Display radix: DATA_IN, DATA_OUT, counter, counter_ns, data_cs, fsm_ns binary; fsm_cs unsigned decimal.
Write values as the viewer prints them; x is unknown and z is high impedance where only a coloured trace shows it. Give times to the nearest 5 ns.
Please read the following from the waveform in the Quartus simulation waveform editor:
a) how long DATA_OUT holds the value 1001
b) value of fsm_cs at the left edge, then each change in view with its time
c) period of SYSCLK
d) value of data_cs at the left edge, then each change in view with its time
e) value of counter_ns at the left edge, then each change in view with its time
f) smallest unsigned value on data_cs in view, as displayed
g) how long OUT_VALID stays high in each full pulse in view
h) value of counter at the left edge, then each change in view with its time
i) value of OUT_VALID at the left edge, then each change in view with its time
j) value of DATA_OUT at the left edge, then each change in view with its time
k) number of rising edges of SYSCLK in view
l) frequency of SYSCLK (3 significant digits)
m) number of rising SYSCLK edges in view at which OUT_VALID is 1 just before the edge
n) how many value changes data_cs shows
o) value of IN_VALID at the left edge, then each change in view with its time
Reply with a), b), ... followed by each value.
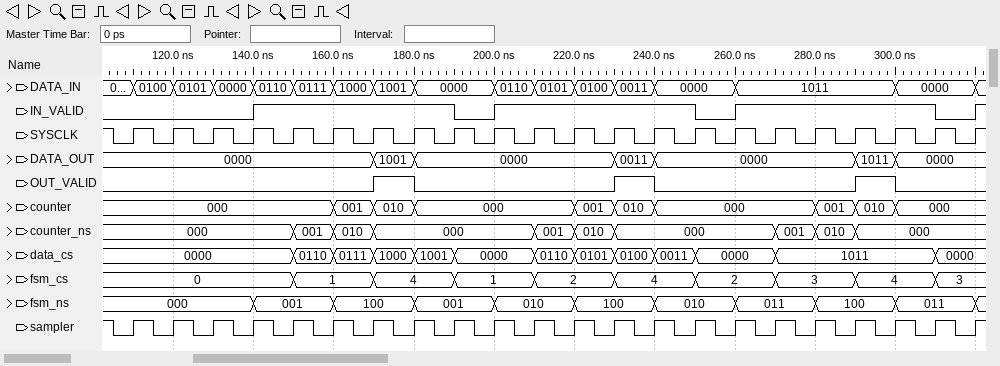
a) 10 ns
b) 0, 1 at 150 ns, 4 at 170 ns, 1 at 190 ns, 2 at 210 ns, 4 at 230 ns, 2 at 250 ns, 3 at 270 ns, 4 at 290 ns, 3 at 310 ns
c) 10 ns
d) 0000, 0110 at 150 ns, 0111 at 160 ns, 1000 at 170 ns, 1001 at 180 ns, 0000 at 190 ns, 0110 at 210 ns, 0101 at 220 ns, 0100 at 230 ns, 0011 at 240 ns, 0000 at 250 ns, 1011 at 270 ns, 0000 at 310 ns
e) 000, 001 at 150 ns, 010 at 160 ns, 000 at 170 ns, 001 at 210 ns, 010 at 220 ns, 000 at 230 ns, 001 at 270 ns, 010 at 280 ns, 000 at 290 ns
f) 0000
g) 10 ns, 10 ns, 10 ns
h) 000, 001 at 160 ns, 010 at 170 ns, 000 at 180 ns, 001 at 220 ns, 010 at 230 ns, 000 at 240 ns, 001 at 280 ns, 010 at 290 ns, 000 at 300 ns
i) 0, 1 at 170 ns, 0 at 180 ns, 1 at 230 ns, 0 at 240 ns, 1 at 290 ns, 0 at 300 ns
j) 0000, 1001 at 170 ns, 0000 at 180 ns, 0011 at 230 ns, 0000 at 240 ns, 1011 at 290 ns, 0000 at 300 ns
k) 22
l) 100 MHz
m) 3
n) 12
o) 0, 1 at 140 ns, 0 at 190 ns, 1 at 200 ns, 0 at 250 ns, 1 at 260 ns, 0 at 310 ns, 1 at 320 ns
